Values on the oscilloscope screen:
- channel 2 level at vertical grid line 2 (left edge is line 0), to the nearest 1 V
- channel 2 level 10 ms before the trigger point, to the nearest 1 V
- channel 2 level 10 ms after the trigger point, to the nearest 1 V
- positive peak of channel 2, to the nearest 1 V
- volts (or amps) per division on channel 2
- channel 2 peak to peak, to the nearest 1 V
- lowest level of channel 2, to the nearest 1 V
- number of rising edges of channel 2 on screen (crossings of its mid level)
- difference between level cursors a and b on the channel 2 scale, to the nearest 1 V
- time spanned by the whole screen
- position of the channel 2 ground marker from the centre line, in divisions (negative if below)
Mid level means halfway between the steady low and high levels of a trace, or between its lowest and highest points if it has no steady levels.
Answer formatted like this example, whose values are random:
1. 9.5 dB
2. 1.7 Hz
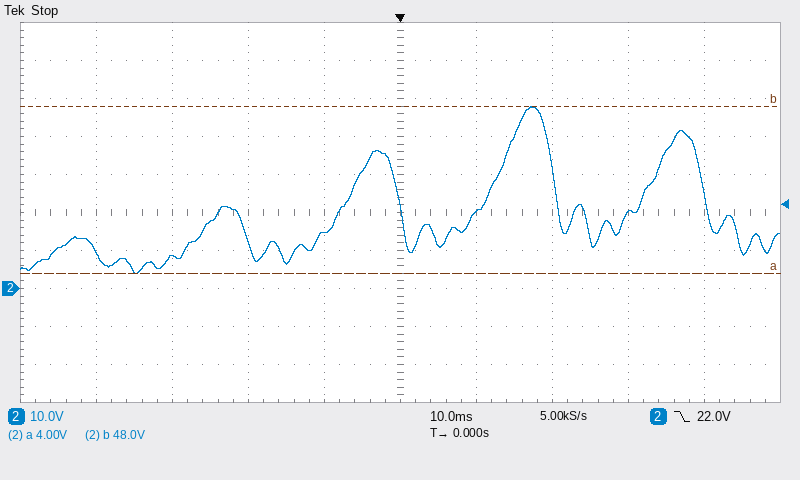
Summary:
1. 8 V
2. 15 V
3. 20 V
4. 48 V
5. 10 V
6. 44 V
7. 4 V
8. 3
9. 44 V
10. 100 ms
11. -2.0 div
